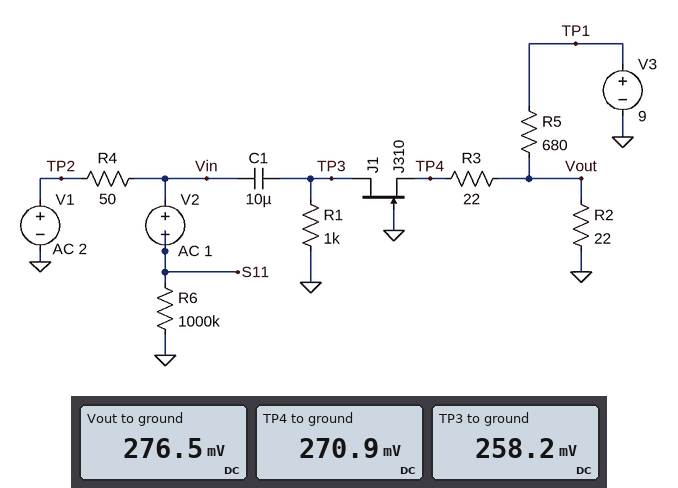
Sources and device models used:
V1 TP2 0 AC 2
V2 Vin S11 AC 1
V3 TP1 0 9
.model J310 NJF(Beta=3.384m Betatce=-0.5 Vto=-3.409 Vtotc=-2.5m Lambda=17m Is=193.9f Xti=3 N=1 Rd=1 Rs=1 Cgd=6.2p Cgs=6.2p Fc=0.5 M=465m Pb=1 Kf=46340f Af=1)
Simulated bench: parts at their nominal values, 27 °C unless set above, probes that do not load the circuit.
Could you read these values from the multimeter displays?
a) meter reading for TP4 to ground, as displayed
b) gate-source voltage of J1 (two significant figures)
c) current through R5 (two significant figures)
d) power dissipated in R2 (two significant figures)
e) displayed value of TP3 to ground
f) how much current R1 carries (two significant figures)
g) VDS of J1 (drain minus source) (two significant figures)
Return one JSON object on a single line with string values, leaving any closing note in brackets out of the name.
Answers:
{"meter reading for TP4 to ground, as displayed": "270.9 mV", "gate-source voltage of J1": "-270 mV", "current through R5": "13 mA", "power dissipated in R2": "3.5 mW", "displayed value of TP3 to ground": "258.2 mV", "how much current R1 carries": "260 µA", "VDS of J1 (drain minus source)": "-13 mV"}
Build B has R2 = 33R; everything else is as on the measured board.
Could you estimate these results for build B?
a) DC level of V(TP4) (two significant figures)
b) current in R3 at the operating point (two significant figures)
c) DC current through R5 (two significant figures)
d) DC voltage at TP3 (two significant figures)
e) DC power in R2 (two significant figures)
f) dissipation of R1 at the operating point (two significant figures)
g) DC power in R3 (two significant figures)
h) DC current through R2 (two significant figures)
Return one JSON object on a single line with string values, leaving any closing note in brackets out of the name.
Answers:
{"DC level of V(TP4)": "400 mV", "current in R3 at the operating point": "380 µA", "DC current through R5": "13 mA", "DC voltage at TP3": "380 mV", "DC power in R2": "5.0 mW", "dissipation of R1 at the operating point": "140 µW", "DC power in R3": "3.1 µW", "DC current through R2": "12 mA"}
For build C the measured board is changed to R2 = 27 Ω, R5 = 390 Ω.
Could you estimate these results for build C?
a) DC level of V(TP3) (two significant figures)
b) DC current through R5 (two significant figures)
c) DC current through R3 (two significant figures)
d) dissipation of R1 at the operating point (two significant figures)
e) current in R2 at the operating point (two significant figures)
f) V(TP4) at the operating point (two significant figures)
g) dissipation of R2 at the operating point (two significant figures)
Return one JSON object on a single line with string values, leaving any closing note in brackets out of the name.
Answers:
{"DC level of V(TP3)": "530 mV", "DC current through R5": "22 mA", "DC current through R3": "530 µA", "dissipation of R1 at the operating point": "280 µW", "current in R2 at the operating point": "21 mA", "V(TP4) at the operating point": "560 mV", "dissipation of R2 at the operating point": "12 mW"}
